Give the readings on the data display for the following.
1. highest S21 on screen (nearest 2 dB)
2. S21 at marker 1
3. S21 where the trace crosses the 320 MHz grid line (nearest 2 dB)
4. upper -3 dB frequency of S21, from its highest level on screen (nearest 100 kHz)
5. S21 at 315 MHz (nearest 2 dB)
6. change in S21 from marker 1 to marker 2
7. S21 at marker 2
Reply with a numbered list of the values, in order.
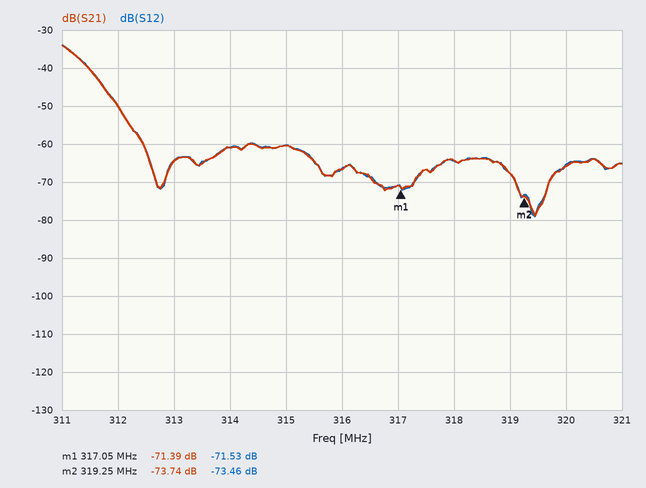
1. -34 dB
2. -71.39 dB
3. -66 dB
4. 311.3 MHz
5. -60 dB
6. -2.35 dB
7. -73.74 dB
